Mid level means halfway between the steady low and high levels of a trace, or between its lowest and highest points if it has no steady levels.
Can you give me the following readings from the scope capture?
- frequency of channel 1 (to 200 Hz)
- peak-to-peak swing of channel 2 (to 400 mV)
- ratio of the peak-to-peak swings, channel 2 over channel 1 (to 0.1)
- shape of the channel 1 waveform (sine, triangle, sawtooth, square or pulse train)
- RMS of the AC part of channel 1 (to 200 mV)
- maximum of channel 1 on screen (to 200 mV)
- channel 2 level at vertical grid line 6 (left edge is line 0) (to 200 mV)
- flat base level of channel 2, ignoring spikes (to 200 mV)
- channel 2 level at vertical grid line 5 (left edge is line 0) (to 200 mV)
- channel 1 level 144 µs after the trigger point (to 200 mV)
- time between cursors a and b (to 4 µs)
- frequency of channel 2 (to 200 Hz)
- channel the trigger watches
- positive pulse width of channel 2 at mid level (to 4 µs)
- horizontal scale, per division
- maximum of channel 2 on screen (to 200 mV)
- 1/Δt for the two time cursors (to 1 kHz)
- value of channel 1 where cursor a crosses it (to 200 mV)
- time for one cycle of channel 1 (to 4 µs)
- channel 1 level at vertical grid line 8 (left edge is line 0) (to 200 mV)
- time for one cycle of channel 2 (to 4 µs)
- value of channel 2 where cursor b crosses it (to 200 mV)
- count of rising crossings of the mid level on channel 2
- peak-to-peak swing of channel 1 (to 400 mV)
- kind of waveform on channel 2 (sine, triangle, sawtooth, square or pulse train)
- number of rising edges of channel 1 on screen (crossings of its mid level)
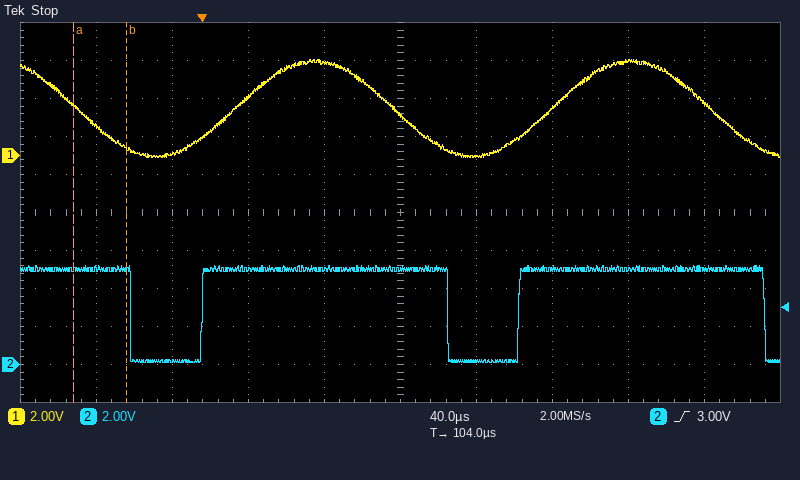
6.0 kHz
5.2 V
1.0
sine
1.8 V
5.0 V
200 mV
200 mV
5.0 V
0.0 V
28 µs
6.0 kHz
channel 2
128 µs
40 µs
5.2 V
36 kHz
2.6 V
168 µs
5.0 V
168 µs
5.0 V
2
5.2 V
pulse train
2
